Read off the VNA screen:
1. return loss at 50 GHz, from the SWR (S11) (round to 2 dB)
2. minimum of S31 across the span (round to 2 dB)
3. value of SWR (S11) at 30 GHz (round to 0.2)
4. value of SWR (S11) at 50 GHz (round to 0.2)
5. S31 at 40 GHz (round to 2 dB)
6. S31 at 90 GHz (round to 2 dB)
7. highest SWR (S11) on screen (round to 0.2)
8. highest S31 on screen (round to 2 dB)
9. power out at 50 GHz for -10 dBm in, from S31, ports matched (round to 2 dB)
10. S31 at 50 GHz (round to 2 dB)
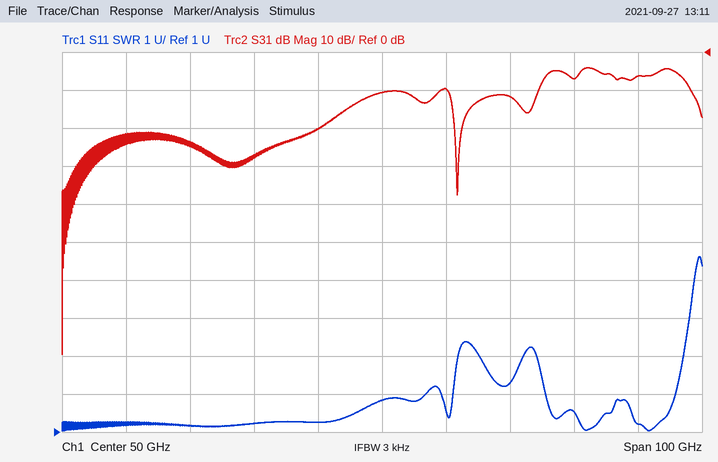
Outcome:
10 dB
-80 dB
1.2
1.8
-20 dB
-6 dB
5.6
-4 dB
-20 dBm
-10 dB
